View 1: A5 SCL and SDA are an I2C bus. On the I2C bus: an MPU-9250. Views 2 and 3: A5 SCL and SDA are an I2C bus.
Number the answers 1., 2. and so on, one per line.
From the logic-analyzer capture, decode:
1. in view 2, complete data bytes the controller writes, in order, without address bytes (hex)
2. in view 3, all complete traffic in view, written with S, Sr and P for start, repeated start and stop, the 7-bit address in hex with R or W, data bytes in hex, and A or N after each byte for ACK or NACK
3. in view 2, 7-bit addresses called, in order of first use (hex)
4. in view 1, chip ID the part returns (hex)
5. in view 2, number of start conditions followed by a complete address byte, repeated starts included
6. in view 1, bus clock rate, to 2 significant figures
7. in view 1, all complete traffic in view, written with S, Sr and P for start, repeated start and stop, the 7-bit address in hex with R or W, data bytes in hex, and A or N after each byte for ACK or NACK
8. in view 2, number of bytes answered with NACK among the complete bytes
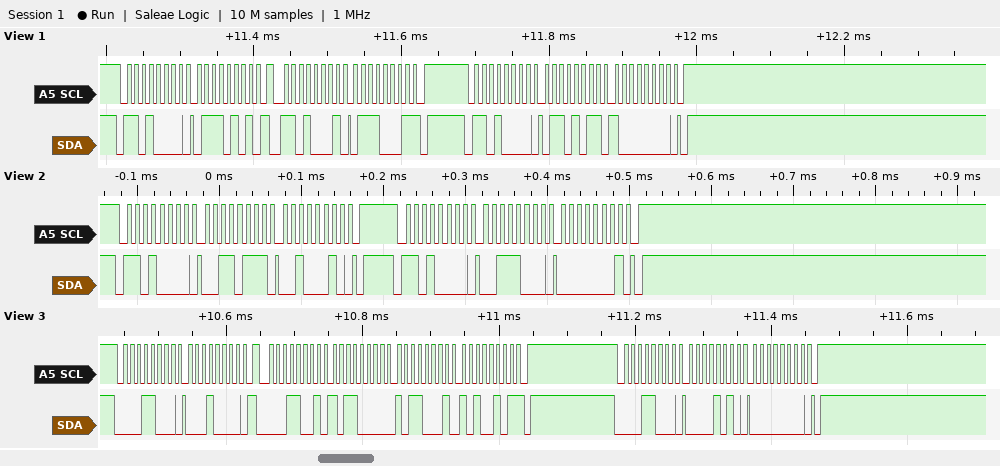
1. 37 22 38 01
2. S 0CW A 10 A Sr 0CR A B0 A B1 A A5 N P S 0CW A 0A A 00 A P
3. 0x68
4. 0x71
5. 2
6. 100 kHz
7. S 68W A 75 A Sr 68R A 71 N P S 68W A 6B A 80 A P
8. 0
